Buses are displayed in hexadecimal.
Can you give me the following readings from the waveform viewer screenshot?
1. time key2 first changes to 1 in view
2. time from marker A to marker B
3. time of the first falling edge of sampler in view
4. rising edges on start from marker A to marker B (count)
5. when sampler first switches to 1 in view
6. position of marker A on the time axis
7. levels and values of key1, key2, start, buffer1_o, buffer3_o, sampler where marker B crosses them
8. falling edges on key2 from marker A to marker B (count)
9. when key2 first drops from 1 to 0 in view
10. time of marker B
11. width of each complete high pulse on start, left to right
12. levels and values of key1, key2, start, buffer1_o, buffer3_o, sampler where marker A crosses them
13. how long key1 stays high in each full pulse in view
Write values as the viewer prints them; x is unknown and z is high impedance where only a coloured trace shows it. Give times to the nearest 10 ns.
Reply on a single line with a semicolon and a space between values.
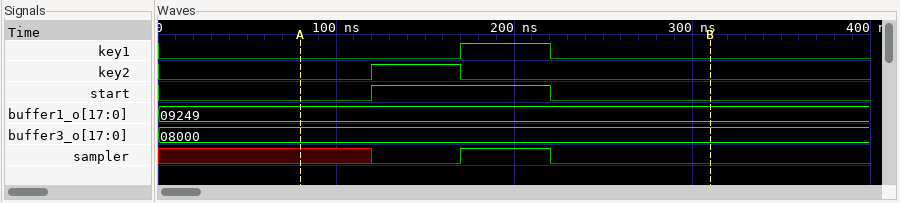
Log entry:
120 ns; 230 ns; 220 ns; 1; 170 ns; 80 ns; key1=0, key2=0, start=0, buffer1_o=09249, buffer3_o=08000, sampler=0; 1; 170 ns; 310 ns; 100 ns; key1=0, key2=0, start=0, buffer1_o=09249, buffer3_o=08000, sampler=x; 50 ns
